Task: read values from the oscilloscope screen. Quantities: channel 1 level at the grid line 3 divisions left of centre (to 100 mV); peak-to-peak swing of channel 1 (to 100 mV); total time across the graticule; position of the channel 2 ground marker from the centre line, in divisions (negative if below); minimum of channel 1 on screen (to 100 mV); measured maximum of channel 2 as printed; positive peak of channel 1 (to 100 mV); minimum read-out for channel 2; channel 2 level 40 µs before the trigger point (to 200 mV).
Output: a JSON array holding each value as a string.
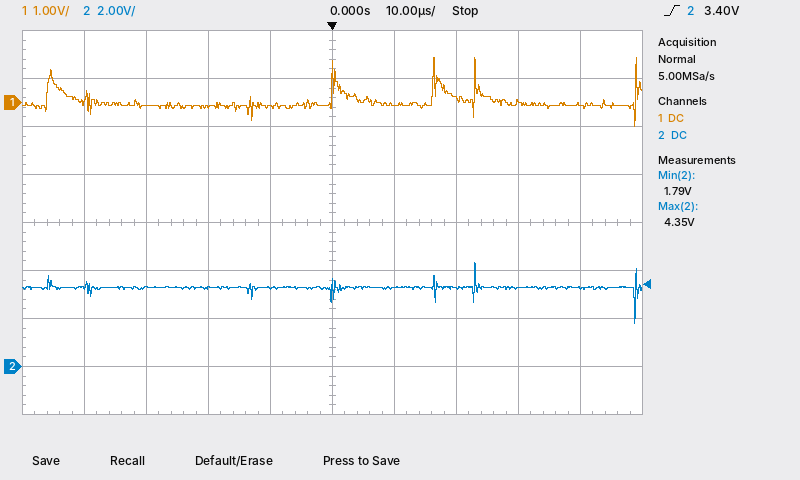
["-100 mV", "1.4 V", "100 µs", "-3.0 div", "-500 mV", "4.35 V", "900 mV", "1.79 V", "3.4 V"]
